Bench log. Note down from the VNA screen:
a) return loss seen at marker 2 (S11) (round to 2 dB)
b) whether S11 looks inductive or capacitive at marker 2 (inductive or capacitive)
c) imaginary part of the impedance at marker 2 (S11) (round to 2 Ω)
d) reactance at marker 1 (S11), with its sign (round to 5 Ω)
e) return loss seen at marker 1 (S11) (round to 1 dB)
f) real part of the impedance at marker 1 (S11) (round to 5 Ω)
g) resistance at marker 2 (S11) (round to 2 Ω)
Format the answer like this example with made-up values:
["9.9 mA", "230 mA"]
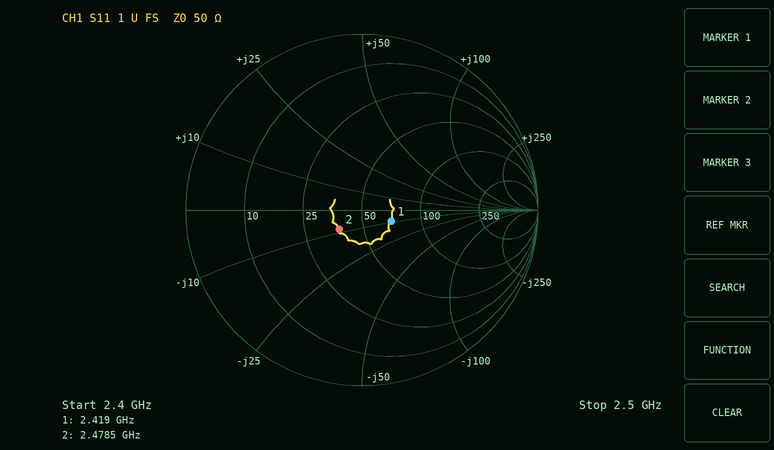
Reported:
["16 dB", "capacitive", "-8 Ω", "-10 Ω", "15 dB", "70 Ω", "38 Ω"]
